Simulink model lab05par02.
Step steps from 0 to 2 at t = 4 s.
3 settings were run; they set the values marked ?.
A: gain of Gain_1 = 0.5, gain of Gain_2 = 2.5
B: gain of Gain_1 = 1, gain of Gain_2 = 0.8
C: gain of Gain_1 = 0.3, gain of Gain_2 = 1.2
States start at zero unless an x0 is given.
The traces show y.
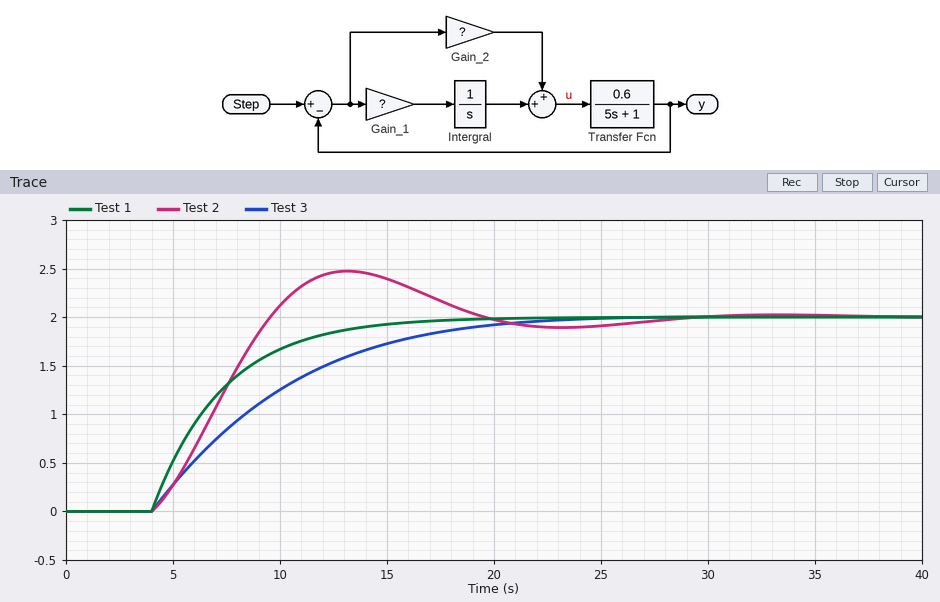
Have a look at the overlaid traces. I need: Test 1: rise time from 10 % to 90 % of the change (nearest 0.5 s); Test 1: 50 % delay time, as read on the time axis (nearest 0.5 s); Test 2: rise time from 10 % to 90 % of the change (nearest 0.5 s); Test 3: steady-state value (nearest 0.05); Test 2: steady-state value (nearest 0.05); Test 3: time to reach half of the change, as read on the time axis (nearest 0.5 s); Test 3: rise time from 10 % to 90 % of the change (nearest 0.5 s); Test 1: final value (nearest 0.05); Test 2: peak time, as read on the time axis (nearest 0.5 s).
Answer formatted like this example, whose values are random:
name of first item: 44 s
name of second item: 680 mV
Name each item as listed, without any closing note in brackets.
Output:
Test 1: rise time from 10 % to 90 % of the change: 7.5 s
Test 1: 50 % delay time, as read on the time axis: 6.5 s
Test 2: rise time from 10 % to 90 % of the change: 4.0 s
Test 3: steady-state value: 2.00
Test 2: steady-state value: 2.00
Test 3: time to reach half of the change, as read on the time axis: 8.5 s
Test 3: rise time from 10 % to 90 % of the change: 11.5 s
Test 1: final value: 2.00
Test 2: peak time, as read on the time axis: 13.0 s
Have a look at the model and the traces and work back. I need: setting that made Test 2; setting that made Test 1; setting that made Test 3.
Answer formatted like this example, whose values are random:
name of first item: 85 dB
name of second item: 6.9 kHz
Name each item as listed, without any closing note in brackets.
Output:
setting that made Test 2: B
setting that made Test 1: A
setting that made Test 3: C
